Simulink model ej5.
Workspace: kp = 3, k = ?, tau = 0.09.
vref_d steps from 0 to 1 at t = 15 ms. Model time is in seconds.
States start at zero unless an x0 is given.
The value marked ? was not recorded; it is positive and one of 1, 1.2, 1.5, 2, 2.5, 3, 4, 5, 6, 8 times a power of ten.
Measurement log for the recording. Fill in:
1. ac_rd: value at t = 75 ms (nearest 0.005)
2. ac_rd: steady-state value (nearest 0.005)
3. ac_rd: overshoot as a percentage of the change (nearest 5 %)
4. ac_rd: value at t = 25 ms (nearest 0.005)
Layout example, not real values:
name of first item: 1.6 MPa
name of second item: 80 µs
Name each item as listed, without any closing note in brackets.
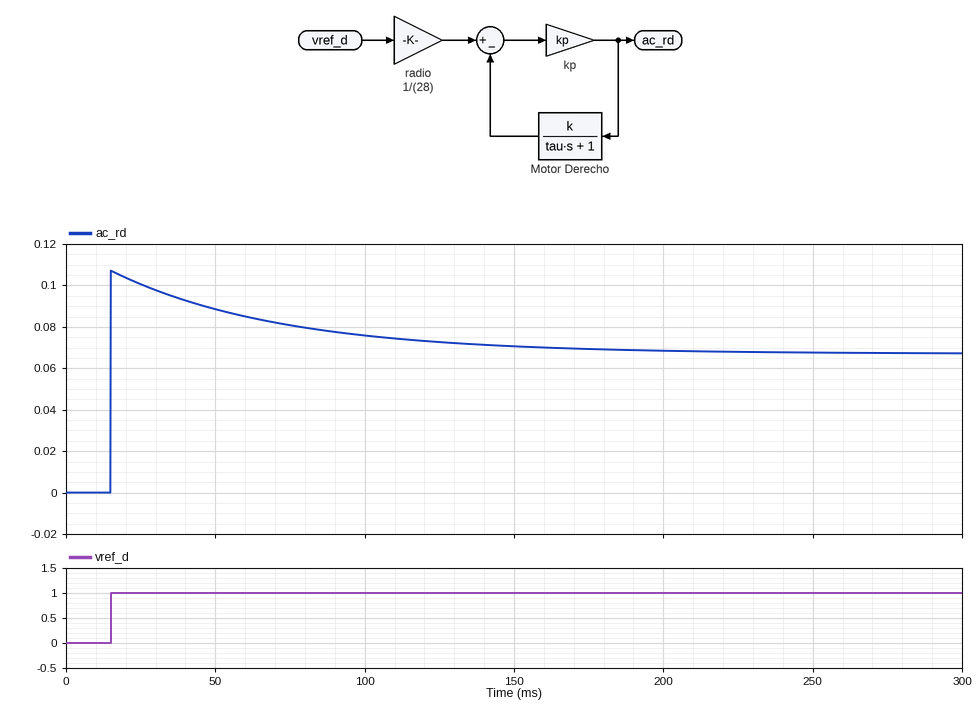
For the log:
ac_rd: value at t = 75 ms: 0.080
ac_rd: steady-state value: 0.065
ac_rd: overshoot as a percentage of the change: 60 %
ac_rd: value at t = 25 ms: 0.100
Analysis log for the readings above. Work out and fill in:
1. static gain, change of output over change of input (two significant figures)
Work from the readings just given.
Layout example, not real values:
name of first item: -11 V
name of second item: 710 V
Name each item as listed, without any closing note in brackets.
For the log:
static gain, change of output over change of input: 0.065
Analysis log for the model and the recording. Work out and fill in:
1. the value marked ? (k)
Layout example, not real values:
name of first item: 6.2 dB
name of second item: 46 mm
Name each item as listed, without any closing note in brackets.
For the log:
the value marked ?: 0.2
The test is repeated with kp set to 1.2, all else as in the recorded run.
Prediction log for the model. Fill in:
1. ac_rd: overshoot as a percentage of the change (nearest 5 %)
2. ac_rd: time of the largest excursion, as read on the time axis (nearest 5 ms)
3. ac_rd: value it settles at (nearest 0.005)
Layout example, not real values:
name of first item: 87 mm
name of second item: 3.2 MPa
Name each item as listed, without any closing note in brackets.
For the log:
ac_rd: overshoot as a percentage of the change: 25 %
ac_rd: time of the largest excursion, as read on the time axis: 15 ms
ac_rd: value it settles at: 0.035
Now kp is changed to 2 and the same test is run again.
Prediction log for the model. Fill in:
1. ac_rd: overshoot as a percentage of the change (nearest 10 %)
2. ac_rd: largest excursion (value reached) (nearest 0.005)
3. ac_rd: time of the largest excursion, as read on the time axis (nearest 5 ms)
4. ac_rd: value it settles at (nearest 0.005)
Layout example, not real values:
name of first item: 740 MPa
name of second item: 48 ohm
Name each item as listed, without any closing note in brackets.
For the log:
ac_rd: overshoot as a percentage of the change: 40 %
ac_rd: largest excursion (value reached): 0.070
ac_rd: time of the largest excursion, as read on the time axis: 15 ms
ac_rd: value it settles at: 0.050
